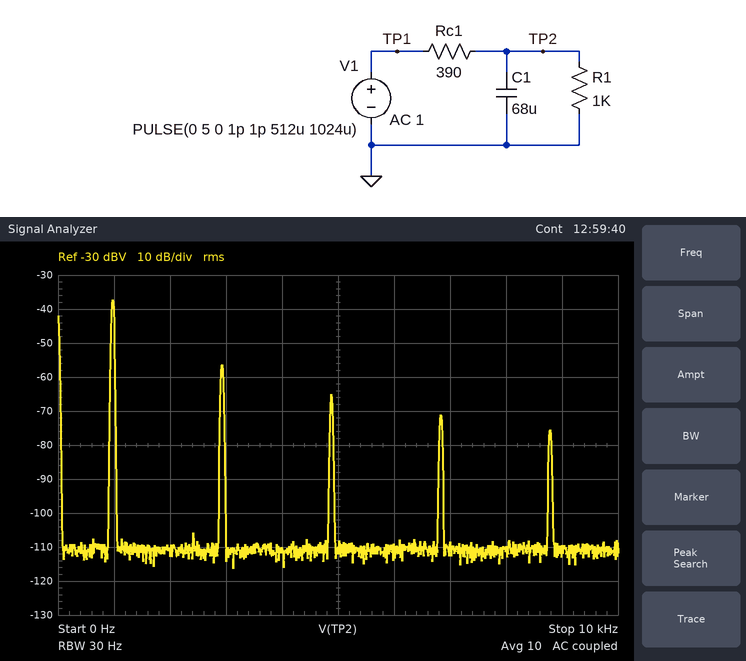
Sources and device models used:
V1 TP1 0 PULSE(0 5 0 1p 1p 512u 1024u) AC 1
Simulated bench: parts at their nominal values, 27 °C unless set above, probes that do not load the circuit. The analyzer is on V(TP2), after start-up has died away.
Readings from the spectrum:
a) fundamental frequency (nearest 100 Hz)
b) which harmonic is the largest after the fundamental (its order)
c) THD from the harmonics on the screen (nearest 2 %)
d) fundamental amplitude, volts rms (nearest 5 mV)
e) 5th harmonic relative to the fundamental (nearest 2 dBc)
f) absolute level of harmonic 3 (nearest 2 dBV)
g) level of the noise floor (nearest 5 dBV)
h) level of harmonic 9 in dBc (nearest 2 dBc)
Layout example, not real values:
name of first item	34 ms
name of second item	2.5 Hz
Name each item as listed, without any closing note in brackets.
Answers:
fundamental frequency	1.0 kHz
which harmonic is the largest after the fundamental	3
THD from the harmonics on the screen	12 %
fundamental amplitude, volts rms	15 mV
5th harmonic relative to the fundamental	-28 dBc
absolute level of harmonic 3	-56 dBV
level of the noise floor	-110 dBV
level of harmonic 9 in dBc	-38 dBc
